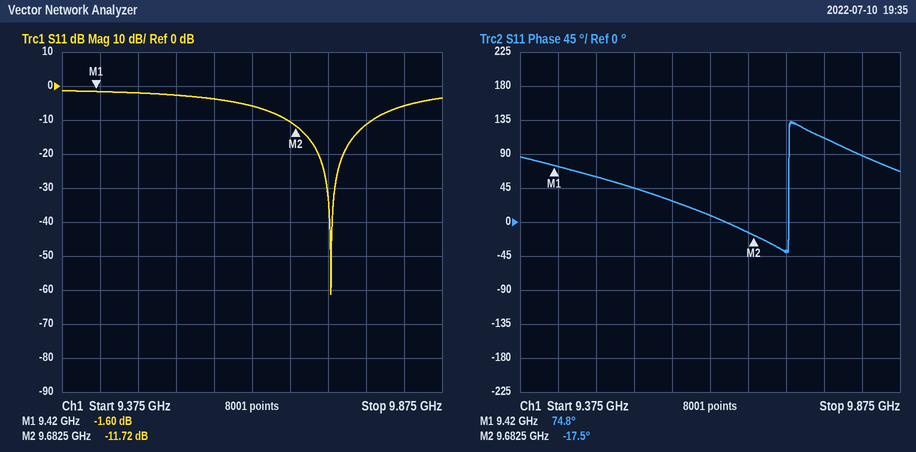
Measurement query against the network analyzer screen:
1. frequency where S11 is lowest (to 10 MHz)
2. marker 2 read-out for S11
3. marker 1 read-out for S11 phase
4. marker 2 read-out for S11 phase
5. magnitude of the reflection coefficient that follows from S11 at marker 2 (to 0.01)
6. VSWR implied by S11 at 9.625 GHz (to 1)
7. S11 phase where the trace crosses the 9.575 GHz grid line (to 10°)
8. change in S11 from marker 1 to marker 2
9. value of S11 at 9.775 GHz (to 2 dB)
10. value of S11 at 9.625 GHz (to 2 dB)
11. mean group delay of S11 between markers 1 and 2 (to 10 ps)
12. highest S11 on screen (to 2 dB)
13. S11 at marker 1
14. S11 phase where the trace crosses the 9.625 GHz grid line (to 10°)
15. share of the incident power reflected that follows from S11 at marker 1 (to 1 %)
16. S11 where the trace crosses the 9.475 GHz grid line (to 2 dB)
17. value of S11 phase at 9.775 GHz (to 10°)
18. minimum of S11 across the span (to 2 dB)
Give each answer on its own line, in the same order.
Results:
9.73 GHz
-11.72 dB
74.8°
-17.5°
0.26
3
30°
-10.12 dB
-12 dB
-6 dB
980 ps
-2 dB
-1.60 dB
10°
69 %
-2 dB
110°
-62 dB
